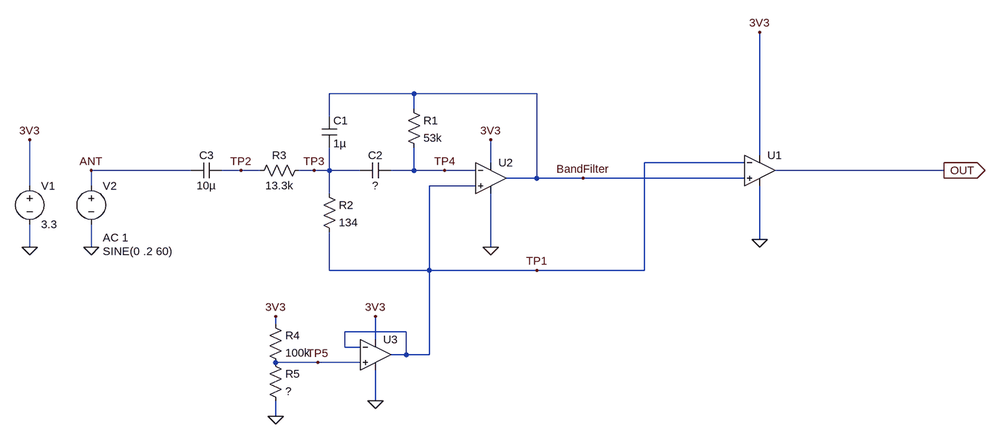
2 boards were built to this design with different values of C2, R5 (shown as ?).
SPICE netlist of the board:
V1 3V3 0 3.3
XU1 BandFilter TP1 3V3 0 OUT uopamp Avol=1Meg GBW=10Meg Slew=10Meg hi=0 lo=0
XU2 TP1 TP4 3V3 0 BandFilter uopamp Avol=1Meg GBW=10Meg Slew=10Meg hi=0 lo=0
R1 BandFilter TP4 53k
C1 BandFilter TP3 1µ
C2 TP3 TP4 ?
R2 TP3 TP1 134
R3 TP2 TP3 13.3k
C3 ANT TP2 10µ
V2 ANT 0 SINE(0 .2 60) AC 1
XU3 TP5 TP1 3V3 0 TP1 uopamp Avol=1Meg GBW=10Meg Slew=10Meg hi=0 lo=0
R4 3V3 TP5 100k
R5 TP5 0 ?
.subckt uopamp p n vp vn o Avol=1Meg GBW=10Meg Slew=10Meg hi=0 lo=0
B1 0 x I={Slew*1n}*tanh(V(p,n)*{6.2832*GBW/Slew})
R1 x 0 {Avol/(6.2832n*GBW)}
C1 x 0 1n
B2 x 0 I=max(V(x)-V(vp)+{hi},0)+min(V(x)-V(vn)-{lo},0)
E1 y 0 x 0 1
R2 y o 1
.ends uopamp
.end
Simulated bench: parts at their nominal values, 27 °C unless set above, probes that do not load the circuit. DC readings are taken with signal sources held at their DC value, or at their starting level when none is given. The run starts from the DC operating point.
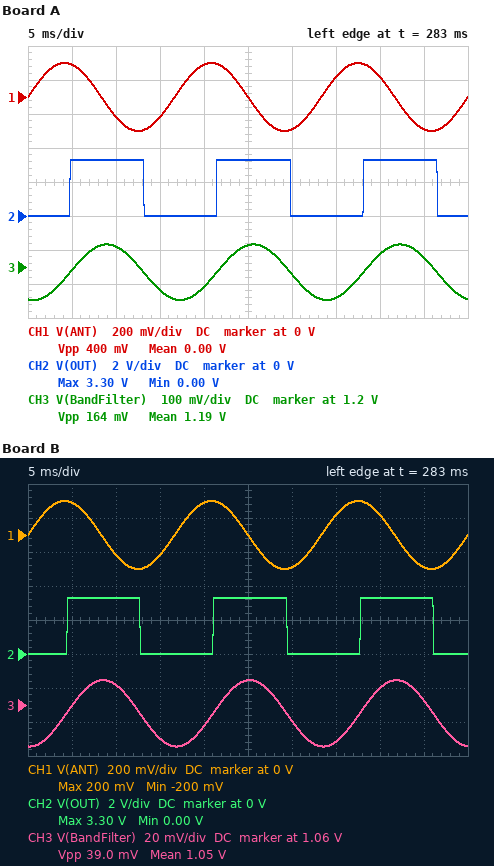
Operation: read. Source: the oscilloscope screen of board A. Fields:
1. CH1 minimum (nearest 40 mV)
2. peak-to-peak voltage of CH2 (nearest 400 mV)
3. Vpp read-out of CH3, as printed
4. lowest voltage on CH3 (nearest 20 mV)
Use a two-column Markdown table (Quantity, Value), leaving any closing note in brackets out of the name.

| Quantity | Value |
|---|---|
| CH1 minimum | -200 mV |
| peak-to-peak voltage of CH2 | 3.2 V |
| Vpp read-out of CH3, as printed | 164 mV |
| lowest voltage on CH3 | 1.10 V |
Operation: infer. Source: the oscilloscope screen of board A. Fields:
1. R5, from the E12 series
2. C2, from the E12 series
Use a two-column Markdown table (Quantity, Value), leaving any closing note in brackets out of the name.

| Quantity | Value |
|---|---|
| R5, from the E12 series | 56 kΩ |
| C2, from the E12 series | 680 nF |
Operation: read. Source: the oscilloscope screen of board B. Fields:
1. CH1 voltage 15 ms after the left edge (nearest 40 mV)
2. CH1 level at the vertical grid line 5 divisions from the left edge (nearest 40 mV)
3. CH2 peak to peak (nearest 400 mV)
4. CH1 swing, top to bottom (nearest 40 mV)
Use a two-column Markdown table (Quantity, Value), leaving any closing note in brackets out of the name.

| Quantity | Value |
|---|---|
| CH1 voltage 15 ms after the left edge | -120 mV |
| CH1 level at the vertical grid line 5 divisions from the left edge | 0 V |
| CH2 peak to peak | 3.2 V |
| CH1 swing, top to bottom | 400 mV |
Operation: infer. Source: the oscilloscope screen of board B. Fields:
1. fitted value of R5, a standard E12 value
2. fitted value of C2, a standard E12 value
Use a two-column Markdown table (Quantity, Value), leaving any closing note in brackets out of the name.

| Quantity | Value |
|---|---|
| fitted value of R5, a standard E12 value | 47 kΩ |
| fitted value of C2, a standard E12 value | 330 nF |
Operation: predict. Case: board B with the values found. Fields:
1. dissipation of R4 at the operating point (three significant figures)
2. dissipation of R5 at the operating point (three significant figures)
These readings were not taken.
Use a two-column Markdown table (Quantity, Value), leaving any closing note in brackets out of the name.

| Quantity | Value |
|---|---|
| dissipation of R4 at the operating point | 50.4 µW |
| dissipation of R5 at the operating point | 23.7 µW |
